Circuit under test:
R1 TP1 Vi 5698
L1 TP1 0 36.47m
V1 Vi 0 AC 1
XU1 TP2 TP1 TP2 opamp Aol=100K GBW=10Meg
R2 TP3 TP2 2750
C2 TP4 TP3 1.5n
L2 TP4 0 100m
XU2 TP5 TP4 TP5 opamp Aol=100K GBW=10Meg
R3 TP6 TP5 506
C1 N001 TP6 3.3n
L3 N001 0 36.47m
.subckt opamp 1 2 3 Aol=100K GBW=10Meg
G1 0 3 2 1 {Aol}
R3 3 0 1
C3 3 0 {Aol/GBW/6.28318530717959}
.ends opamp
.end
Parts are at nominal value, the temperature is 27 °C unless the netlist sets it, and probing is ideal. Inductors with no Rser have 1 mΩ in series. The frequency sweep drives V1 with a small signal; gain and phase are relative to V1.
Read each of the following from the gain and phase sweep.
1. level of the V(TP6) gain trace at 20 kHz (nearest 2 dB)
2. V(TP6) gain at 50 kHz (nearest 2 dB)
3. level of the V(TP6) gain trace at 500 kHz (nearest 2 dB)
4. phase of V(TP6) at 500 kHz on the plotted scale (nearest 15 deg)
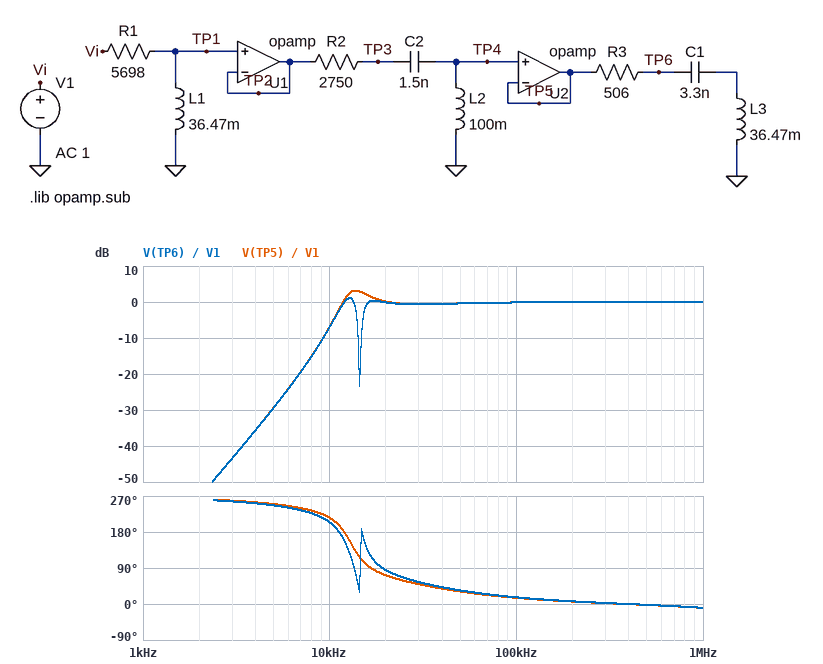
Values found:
0 dB
0 dB
0 dB
0 deg
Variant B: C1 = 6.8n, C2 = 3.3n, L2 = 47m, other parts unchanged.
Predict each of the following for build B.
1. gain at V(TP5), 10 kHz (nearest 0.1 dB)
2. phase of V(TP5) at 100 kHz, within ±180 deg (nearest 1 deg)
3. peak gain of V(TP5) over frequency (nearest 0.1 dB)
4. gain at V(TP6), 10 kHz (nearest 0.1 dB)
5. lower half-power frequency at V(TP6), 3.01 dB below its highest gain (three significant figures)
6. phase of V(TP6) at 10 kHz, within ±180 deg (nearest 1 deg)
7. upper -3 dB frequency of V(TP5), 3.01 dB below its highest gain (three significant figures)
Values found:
-9.6 dB
18 deg
0 dB
-29.9 dB
14.4 kHz
108 deg
6.47 MHz
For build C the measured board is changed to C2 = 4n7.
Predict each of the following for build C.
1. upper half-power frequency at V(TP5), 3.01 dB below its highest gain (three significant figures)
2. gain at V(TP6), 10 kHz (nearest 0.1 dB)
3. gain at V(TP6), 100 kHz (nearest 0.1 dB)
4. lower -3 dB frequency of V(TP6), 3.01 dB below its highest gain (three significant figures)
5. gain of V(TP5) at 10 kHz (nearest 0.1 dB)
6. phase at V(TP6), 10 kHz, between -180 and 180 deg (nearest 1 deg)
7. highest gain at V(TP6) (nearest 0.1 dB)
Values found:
6.47 MHz
-4.8 dB
-0.2 dB
21.2 kHz
-4.6 dB
100 deg
0 dB
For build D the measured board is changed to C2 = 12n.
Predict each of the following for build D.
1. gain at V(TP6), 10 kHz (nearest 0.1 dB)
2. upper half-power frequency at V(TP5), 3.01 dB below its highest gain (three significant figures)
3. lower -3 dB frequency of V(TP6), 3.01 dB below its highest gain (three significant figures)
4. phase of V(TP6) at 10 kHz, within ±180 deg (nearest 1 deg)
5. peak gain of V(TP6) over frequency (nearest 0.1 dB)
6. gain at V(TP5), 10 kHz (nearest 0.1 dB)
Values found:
-7.8 dB
6.47 MHz
24.2 kHz
86 deg
0 dB
-7.7 dB
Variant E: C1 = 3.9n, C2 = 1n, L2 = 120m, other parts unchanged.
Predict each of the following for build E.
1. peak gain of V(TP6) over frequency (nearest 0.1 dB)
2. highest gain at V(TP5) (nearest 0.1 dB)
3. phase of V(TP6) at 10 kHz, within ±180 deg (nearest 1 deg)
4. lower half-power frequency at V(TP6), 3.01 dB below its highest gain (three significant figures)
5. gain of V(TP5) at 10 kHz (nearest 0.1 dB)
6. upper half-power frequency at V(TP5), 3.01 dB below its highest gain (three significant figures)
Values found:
4.9 dB
6.3 dB
-146 deg
14.3 kHz
-9.9 dB
18.0 kHz
